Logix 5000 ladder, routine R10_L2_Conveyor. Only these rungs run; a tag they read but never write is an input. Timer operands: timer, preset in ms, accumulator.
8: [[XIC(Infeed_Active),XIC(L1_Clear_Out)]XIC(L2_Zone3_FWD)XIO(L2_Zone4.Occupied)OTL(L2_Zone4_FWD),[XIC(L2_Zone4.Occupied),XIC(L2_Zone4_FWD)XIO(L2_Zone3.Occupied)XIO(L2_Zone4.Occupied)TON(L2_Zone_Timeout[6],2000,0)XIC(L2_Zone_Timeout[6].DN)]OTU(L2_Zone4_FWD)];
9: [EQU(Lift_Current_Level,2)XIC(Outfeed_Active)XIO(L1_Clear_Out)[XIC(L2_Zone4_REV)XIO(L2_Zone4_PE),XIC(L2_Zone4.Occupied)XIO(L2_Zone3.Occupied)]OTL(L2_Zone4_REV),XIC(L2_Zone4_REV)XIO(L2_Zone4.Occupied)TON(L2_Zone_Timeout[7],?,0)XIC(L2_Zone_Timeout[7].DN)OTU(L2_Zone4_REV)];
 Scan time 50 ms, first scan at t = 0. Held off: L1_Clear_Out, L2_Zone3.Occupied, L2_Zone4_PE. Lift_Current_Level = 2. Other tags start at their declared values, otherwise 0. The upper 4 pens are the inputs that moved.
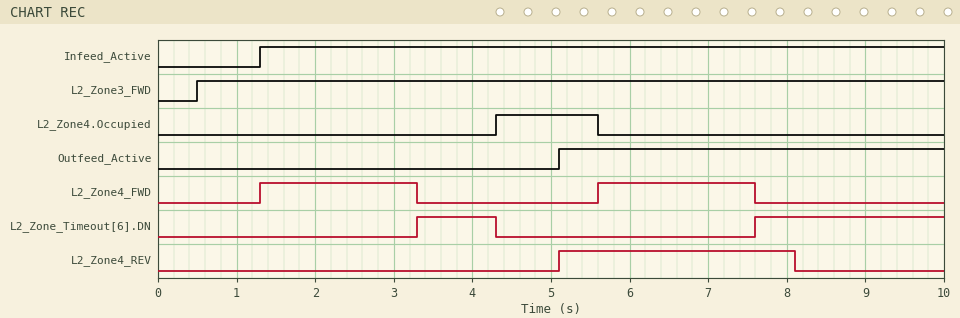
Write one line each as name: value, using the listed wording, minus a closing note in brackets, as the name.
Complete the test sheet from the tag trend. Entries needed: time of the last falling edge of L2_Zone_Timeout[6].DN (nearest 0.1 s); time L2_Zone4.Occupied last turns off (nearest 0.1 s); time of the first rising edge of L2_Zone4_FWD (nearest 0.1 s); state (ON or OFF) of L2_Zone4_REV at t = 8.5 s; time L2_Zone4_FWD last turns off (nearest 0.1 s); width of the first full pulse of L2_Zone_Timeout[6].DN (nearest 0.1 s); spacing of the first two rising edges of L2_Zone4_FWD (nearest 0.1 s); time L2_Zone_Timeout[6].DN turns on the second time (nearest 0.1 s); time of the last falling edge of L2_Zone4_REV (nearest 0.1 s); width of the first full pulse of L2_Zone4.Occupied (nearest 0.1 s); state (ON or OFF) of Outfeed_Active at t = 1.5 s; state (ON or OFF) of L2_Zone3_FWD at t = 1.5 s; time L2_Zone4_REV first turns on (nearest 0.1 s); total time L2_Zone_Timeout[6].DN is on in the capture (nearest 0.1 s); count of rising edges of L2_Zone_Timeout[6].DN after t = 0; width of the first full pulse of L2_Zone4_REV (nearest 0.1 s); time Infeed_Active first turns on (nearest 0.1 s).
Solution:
time of the last falling edge of L2_Zone_Timeout[6].DN: 4.3 s
time L2_Zone4.Occupied last turns off: 5.6 s
time of the first rising edge of L2_Zone4_FWD: 1.3 s
state (ON or OFF) of L2_Zone4_REV at t = 8.5 s: OFF
time L2_Zone4_FWD last turns off: 7.6 s
width of the first full pulse of L2_Zone_Timeout[6].DN: 1.0 s
spacing of the first two rising edges of L2_Zone4_FWD: 4.3 s
time L2_Zone_Timeout[6].DN turns on the second time: 7.6 s
time of the last falling edge of L2_Zone4_REV: 8.1 s
width of the first full pulse of L2_Zone4.Occupied: 1.3 s
state (ON or OFF) of Outfeed_Active at t = 1.5 s: OFF
state (ON or OFF) of L2_Zone3_FWD at t = 1.5 s: ON
time L2_Zone4_REV first turns on: 5.1 s
total time L2_Zone_Timeout[6].DN is on in the capture: 3.4 s
count of rising edges of L2_Zone_Timeout[6].DN after t = 0: 2
width of the first full pulse of L2_Zone4_REV: 3.0 s
time Infeed_Active first turns on: 1.3 s
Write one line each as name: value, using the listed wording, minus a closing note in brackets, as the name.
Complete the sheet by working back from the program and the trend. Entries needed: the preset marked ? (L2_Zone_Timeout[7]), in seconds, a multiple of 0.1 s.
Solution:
the preset marked ? (L2_Zone_Timeout[7]), in seconds, a multiple of 0.1 s: 2.5 s
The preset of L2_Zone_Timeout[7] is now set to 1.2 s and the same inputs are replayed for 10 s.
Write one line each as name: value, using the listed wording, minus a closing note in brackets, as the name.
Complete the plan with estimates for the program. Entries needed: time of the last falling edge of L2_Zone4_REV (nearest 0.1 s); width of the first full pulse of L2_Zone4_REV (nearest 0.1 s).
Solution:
time of the last falling edge of L2_Zone4_REV: 6.8 s
width of the first full pulse of L2_Zone4_REV: 1.7 s
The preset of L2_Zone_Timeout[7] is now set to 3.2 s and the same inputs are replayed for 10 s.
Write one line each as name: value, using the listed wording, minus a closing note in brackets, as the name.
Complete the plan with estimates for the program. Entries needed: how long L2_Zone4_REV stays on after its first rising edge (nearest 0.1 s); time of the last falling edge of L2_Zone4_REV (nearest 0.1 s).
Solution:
how long L2_Zone4_REV stays on after its first rising edge: 3.7 s
time of the last falling edge of L2_Zone4_REV: 8.8 s
